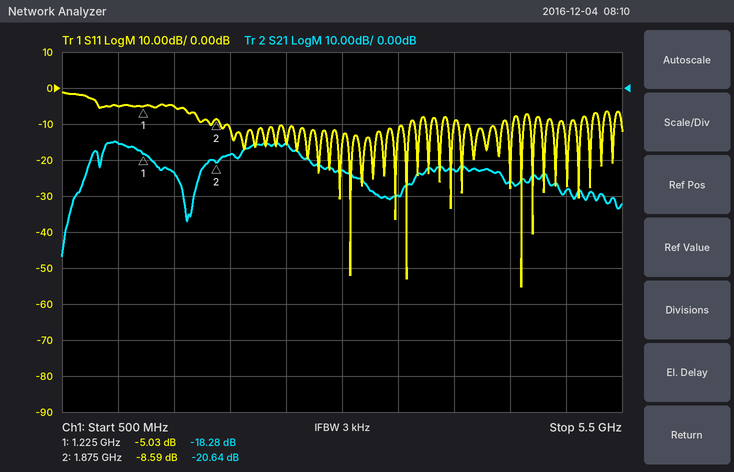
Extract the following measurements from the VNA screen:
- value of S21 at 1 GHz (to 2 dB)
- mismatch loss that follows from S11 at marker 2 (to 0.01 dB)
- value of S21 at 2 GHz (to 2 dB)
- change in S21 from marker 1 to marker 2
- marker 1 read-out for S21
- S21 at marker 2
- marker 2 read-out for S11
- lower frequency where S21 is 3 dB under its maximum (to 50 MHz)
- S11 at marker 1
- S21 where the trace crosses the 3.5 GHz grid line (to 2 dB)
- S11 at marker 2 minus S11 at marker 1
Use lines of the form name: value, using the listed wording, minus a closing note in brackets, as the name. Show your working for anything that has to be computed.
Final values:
value of S21 at 1 GHz: -16 dB
mismatch loss that follows from S11 at marker 2: −10 log10(1 − 10^(-8.59/10)) ≈ 0.65 dB
value of S21 at 2 GHz: -18 dB
change in S21 from marker 1 to marker 2: -20.64 − (-18.28) = -2.36 dB
marker 1 read-out for S21: -18.28 dB
S21 at marker 2: -20.64 dB
marker 2 read-out for S11: -8.59 dB
lower frequency where S21 is 3 dB under its maximum: 850 MHz
S11 at marker 1: -5.03 dB
S21 where the trace crosses the 3.5 GHz grid line: -30 dB
S11 at marker 2 minus S11 at marker 1: -8.59 − (-5.03) = -3.56 dB
